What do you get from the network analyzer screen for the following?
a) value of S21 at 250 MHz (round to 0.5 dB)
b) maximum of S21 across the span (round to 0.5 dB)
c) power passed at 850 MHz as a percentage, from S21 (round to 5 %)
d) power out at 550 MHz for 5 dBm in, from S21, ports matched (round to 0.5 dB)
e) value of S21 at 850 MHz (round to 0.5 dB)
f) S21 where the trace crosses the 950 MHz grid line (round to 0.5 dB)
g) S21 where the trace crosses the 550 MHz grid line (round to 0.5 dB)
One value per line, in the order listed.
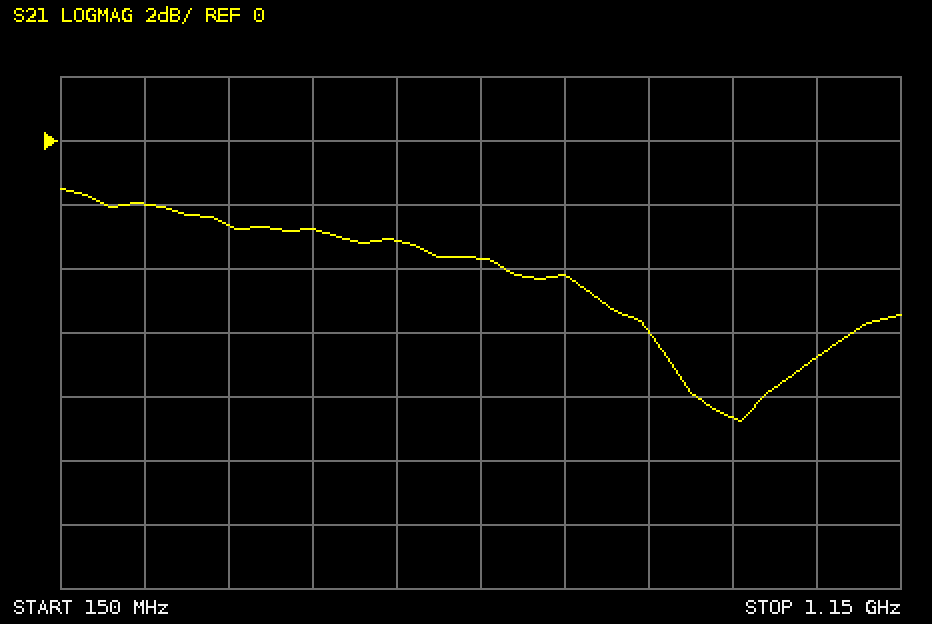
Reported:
-2.0 dB
-1.5 dB
25 %
2.0 dBm
-6.0 dB
-8.5 dB
-3.0 dB
